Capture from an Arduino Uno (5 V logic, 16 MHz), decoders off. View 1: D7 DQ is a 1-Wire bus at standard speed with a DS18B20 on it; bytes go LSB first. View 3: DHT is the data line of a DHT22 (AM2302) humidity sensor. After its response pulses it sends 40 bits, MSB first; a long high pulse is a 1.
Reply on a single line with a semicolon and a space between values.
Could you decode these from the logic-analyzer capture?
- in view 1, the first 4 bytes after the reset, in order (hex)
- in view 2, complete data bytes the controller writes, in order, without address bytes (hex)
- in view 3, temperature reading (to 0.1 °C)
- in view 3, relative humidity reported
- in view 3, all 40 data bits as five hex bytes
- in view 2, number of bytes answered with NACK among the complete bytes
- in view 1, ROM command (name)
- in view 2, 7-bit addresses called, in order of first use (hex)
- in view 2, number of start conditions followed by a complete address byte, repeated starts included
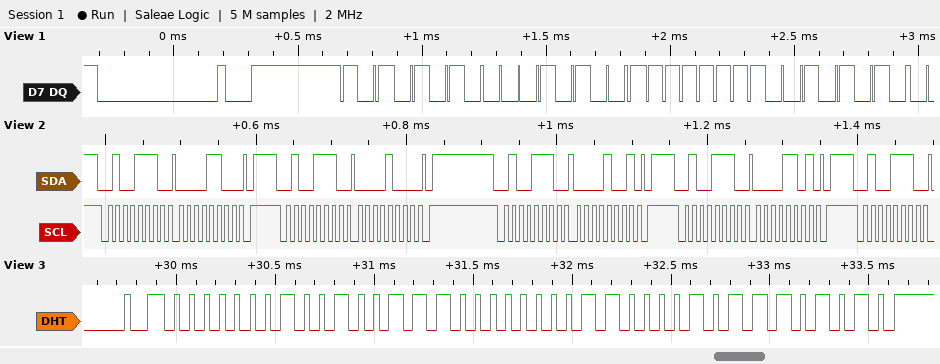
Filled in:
55 28 FF 54; 0C 08 09 0D; 19.4 °C; 29.5 %; 01 27 00 C2 EA; 0; Match ROM; 0x27; 5
